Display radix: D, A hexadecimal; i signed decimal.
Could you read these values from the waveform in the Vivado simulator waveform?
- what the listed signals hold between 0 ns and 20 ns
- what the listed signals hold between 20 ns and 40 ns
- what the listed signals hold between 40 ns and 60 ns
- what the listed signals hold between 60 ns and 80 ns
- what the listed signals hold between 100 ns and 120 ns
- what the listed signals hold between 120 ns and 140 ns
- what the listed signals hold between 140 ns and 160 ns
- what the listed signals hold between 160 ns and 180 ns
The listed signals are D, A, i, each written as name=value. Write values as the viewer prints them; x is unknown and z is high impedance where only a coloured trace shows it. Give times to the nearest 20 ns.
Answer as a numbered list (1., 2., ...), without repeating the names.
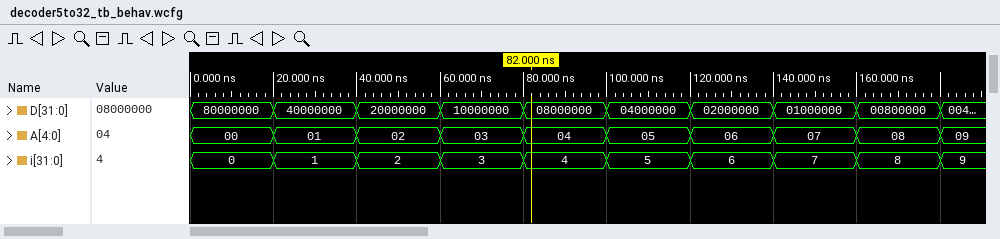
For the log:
1. D=80000000, A=00, i=0
2. D=40000000, A=01, i=1
3. D=20000000, A=02, i=2
4. D=10000000, A=03, i=3
5. D=04000000, A=05, i=5
6. D=02000000, A=06, i=6
7. D=01000000, A=07, i=7
8. D=00800000, A=08, i=8
